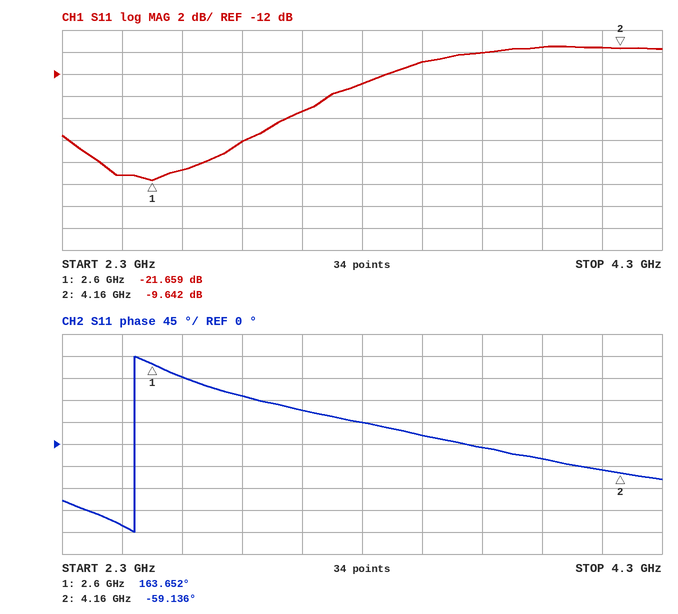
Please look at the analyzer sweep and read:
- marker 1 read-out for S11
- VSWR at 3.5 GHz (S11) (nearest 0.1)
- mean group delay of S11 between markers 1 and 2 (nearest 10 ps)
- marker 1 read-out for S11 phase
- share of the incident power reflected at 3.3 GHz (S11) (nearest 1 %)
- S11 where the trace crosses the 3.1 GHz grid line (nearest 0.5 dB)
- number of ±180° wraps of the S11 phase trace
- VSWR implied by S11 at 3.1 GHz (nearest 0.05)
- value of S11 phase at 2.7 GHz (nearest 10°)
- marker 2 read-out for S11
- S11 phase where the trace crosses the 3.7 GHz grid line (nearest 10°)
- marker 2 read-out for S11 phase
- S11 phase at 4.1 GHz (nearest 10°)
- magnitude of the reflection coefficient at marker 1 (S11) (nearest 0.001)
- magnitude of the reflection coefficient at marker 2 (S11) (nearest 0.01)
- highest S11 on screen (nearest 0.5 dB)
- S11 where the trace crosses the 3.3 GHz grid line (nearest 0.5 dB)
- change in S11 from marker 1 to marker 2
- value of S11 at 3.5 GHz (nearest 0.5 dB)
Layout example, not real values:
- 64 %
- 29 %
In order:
- -21.659 dB
- 1.8
- 400 ps
- 163.652°
- 5 %
- -15.5 dB
- 1
- 1.40
- 140°
- -9.642 dB
- -10°
- -59.136°
- -50°
- 0.083
- 0.33
- -9.5 dB
- -13.0 dB
- 12.017 dB
- -11.0 dB
